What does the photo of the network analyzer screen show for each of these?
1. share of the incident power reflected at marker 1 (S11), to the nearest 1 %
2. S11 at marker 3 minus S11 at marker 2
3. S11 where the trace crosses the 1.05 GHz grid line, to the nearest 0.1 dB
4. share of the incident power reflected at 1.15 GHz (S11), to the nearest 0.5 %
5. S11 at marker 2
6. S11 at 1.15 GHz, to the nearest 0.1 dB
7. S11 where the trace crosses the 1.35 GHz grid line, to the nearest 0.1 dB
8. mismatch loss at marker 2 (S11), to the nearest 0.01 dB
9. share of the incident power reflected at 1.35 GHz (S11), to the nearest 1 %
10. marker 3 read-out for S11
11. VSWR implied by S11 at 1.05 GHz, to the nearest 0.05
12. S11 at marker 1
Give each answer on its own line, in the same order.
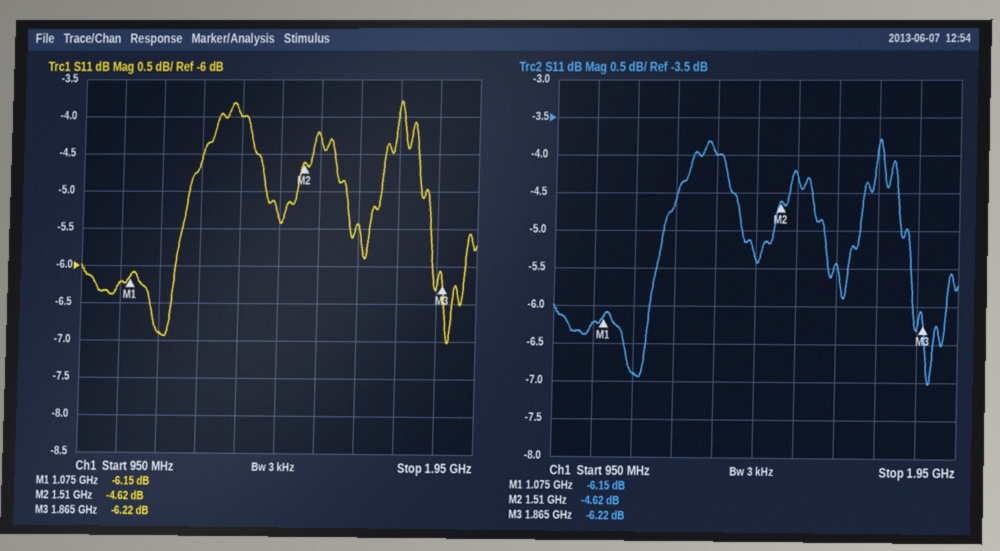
24 %
-1.60 dB
-6.2 dB
20.5 %
-4.62 dB
-6.9 dB
-4.0 dB
1.84 dB
40 %
-6.22 dB
2.90
-6.15 dB
